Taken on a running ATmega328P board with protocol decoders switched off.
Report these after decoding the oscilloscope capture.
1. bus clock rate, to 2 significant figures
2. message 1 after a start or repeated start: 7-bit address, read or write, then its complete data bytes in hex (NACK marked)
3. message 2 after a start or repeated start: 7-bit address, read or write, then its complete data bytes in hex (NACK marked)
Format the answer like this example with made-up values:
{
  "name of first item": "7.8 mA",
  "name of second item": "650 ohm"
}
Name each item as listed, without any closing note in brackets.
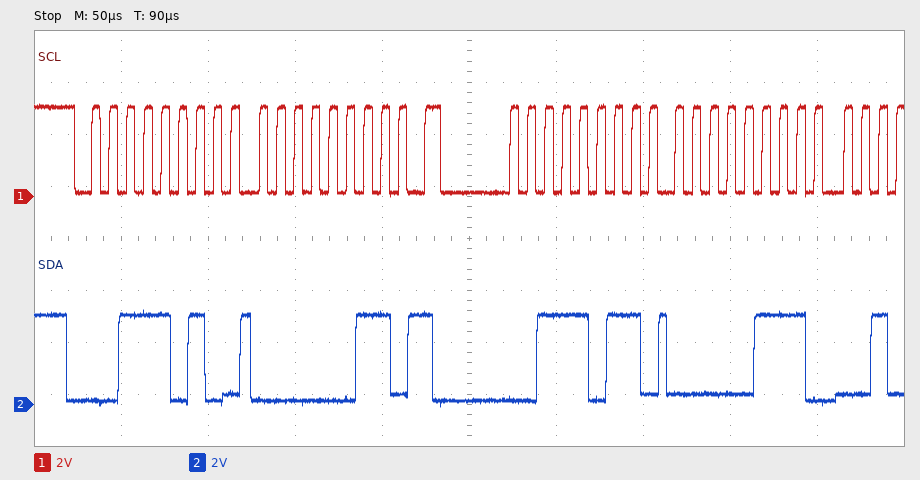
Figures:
{
  "bus clock rate, to 2 significant figures": "100 kHz",
  "message 1 after a start or repeated start: 7-bit address, read or write, then its complete data bytes in hex": "0x1D write: 03",
  "message 2 after a start or repeated start: 7-bit address, read or write, then its complete data bytes in hex": "0x1D read: 07"
}
